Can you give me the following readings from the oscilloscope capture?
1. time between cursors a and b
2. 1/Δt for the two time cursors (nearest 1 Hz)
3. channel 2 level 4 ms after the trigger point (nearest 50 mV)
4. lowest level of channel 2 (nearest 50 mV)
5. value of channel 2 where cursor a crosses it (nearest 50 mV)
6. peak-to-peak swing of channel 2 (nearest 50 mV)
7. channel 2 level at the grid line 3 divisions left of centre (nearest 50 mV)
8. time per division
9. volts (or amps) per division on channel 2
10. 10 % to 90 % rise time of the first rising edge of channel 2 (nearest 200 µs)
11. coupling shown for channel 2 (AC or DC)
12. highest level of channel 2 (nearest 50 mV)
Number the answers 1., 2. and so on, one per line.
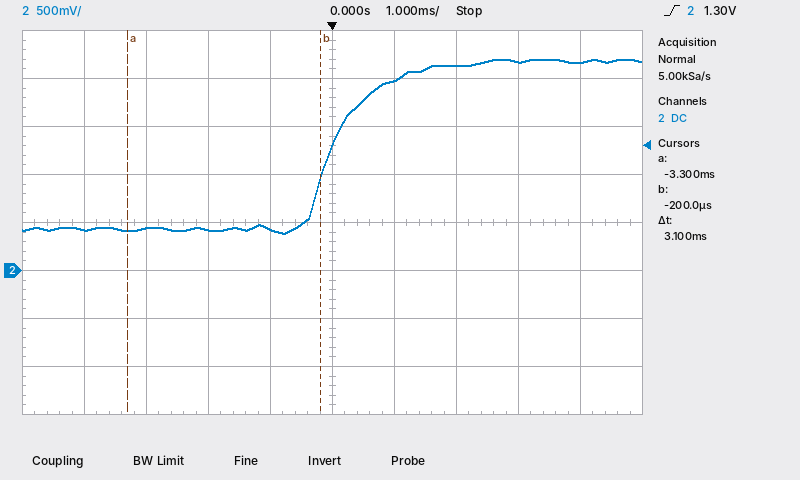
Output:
1. 3.1 ms
2. 323 Hz
3. 2.15 V
4. 400 mV
5. 400 mV
6. 1.80 V
7. 450 mV
8. 1 ms
9. 500 mV
10. 1.4 ms
11. DC
12. 2.20 V
